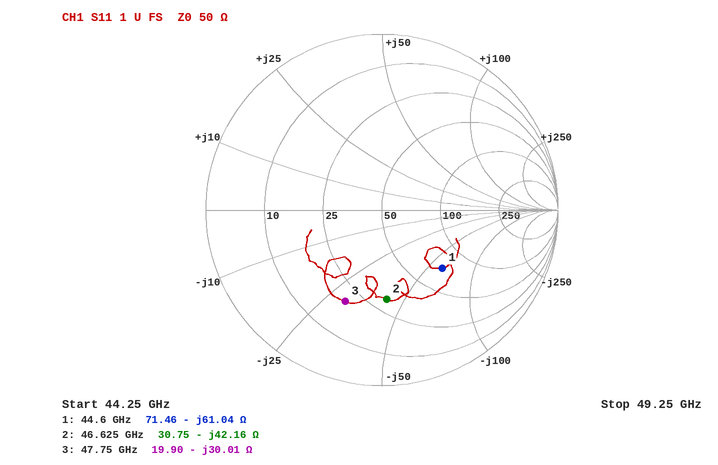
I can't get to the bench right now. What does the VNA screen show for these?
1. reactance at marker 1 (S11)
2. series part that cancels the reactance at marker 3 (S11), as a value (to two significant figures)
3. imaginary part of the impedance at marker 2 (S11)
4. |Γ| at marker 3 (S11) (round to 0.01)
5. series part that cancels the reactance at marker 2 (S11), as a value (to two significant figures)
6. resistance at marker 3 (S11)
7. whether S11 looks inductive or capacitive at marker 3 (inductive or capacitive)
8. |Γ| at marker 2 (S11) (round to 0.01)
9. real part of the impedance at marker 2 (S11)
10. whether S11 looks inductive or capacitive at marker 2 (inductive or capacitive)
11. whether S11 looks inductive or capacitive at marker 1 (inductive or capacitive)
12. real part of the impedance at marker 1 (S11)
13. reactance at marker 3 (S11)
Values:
-61.04 Ω
100 pH
-42.16 Ω
0.56
140 pH
19.90 Ω
capacitive
0.51
30.75 Ω
capacitive
capacitive
71.46 Ω
-30.01 Ω
